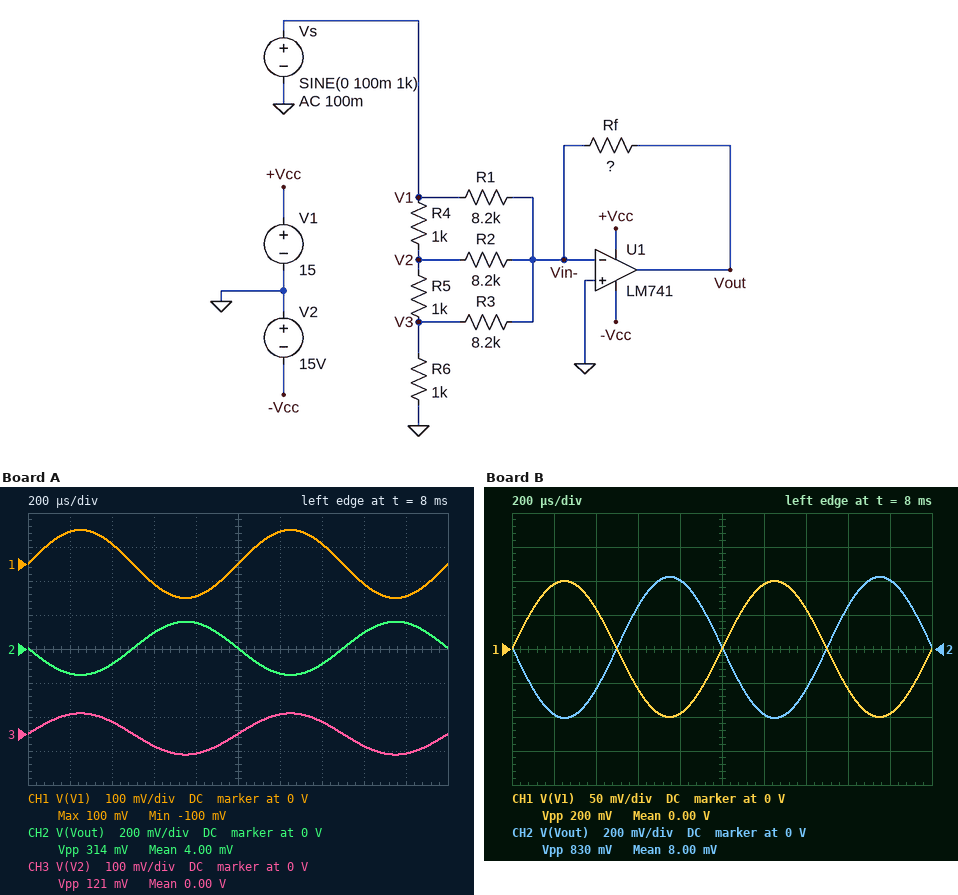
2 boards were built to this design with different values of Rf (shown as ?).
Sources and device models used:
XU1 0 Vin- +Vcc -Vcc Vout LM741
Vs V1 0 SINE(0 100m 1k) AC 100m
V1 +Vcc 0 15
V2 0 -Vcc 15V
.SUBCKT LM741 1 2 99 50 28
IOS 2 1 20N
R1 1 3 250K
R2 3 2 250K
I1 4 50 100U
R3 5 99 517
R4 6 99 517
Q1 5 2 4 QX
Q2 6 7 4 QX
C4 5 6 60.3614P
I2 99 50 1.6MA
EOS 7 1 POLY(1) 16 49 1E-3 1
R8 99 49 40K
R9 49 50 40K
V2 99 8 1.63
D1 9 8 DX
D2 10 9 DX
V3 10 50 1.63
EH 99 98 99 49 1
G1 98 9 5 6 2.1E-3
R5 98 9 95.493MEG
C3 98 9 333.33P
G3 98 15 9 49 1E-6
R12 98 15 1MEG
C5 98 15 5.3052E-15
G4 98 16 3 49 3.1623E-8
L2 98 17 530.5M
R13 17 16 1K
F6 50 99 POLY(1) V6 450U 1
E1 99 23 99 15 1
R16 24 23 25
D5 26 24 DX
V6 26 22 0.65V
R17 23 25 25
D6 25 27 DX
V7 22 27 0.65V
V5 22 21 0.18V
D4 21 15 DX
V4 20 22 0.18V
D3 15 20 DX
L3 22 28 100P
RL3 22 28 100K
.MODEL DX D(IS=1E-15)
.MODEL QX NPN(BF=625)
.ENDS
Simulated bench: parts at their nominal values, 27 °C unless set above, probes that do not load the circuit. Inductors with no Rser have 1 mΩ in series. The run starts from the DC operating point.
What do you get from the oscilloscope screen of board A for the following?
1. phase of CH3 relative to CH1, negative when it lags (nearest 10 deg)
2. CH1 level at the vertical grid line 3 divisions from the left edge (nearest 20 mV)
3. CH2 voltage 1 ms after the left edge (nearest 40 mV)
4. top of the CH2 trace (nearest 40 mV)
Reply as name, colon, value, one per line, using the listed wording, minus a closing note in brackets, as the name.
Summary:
phase of CH3 relative to CH1, negative when it lags: 0 deg
CH1 level at the vertical grid line 3 divisions from the left edge: -60 mV
CH2 voltage 1 ms after the left edge: 0 V
top of the CH2 trace: 160 mV
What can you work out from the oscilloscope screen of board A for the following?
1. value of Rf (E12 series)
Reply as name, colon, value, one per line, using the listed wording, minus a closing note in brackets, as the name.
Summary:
value of Rf: 6.8 kΩ
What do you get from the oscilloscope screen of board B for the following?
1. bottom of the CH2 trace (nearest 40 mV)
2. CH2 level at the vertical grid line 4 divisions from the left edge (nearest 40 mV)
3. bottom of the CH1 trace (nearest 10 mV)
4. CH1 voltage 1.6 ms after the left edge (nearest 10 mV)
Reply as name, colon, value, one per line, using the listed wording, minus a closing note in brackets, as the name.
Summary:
bottom of the CH2 trace: -400 mV
CH2 level at the vertical grid line 4 divisions from the left edge: 400 mV
bottom of the CH1 trace: -100 mV
CH1 voltage 1.6 ms after the left edge: -60 mV
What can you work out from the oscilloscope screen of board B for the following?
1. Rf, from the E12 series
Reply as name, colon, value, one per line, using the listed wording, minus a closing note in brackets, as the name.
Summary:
Rf, from the E12 series: 18 kΩ
